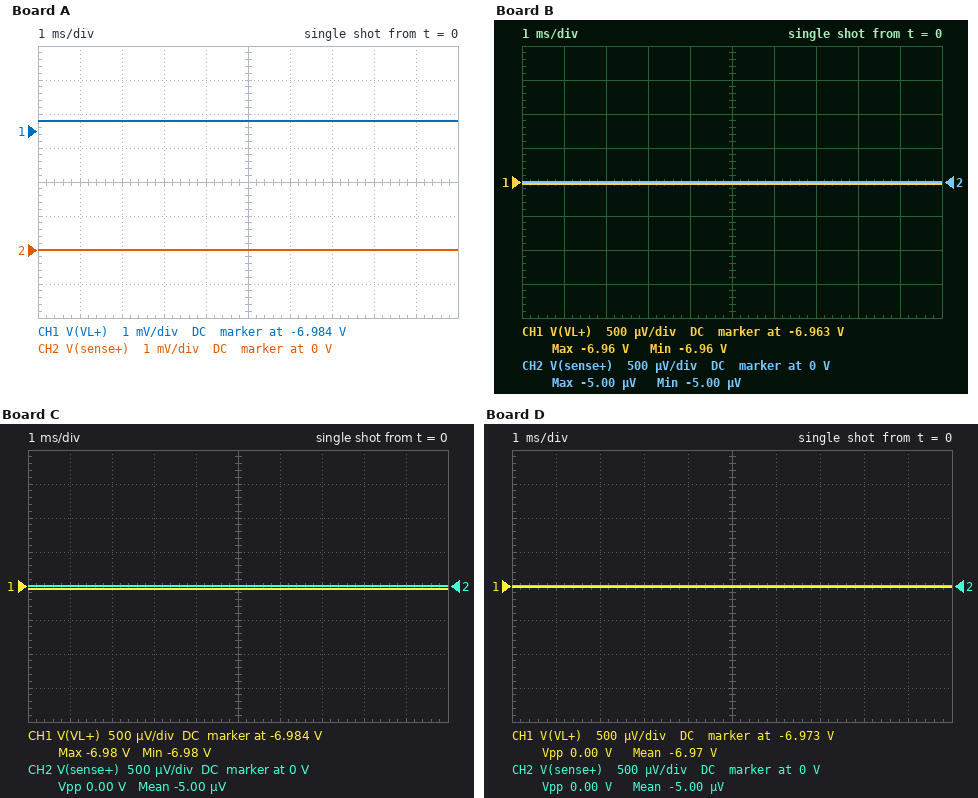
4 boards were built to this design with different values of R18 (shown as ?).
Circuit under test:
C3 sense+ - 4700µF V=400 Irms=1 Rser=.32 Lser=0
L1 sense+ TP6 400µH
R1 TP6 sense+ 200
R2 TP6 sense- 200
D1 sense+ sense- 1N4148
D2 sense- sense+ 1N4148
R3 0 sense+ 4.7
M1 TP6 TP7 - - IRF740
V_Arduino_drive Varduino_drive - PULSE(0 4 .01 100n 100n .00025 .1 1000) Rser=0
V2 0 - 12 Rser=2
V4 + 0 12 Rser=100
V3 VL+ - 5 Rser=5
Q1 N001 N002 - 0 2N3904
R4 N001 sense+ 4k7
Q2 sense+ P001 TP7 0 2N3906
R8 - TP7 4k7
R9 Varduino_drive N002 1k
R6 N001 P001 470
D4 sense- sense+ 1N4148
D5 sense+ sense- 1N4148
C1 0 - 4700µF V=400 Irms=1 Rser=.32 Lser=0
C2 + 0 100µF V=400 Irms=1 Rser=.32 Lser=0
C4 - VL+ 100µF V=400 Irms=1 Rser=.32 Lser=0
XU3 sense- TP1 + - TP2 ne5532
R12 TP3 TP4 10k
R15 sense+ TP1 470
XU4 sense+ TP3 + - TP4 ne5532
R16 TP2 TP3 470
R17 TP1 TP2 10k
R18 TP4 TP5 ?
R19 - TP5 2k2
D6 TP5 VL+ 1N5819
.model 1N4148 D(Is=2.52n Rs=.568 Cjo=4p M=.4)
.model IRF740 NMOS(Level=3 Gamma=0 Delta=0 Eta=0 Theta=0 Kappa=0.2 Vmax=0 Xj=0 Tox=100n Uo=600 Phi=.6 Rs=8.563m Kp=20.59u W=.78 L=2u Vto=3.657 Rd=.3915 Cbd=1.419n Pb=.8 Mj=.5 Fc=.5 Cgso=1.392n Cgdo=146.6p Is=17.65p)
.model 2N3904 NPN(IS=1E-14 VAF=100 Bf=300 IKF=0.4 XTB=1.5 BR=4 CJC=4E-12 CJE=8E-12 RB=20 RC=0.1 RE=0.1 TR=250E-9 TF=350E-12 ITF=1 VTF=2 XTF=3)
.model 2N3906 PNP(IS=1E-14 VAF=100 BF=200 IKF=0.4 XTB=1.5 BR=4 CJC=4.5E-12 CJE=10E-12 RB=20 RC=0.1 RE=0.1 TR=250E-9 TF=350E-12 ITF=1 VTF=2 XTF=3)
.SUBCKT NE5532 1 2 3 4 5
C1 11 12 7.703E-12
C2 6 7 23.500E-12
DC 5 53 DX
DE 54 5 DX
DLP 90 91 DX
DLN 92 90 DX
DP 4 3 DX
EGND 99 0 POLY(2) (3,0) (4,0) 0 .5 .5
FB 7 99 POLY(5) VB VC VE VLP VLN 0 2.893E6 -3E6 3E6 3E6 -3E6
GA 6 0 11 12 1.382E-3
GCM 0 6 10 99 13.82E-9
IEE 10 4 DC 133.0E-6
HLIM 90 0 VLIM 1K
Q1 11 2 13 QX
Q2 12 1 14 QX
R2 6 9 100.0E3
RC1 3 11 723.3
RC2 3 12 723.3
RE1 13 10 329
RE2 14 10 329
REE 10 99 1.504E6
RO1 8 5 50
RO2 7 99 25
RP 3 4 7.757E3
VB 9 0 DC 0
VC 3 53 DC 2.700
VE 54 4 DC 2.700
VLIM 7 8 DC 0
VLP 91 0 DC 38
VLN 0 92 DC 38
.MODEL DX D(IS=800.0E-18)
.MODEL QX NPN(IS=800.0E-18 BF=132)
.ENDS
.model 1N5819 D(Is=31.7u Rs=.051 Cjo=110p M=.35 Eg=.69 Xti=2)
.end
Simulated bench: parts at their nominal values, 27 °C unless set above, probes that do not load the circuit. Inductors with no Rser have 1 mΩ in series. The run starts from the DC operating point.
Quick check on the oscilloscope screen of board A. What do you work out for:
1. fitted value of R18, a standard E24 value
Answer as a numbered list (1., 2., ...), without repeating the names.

1. 3.9 kΩ
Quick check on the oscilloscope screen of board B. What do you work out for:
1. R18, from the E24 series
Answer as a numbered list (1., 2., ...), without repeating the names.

1. 1.3 kΩ
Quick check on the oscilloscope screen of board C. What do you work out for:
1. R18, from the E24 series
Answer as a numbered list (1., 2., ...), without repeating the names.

1. 5.6 kΩ
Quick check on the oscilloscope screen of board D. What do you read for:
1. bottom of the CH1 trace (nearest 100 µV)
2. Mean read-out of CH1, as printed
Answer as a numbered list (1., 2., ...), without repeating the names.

1. -6.9725 V
2. -6.97 V
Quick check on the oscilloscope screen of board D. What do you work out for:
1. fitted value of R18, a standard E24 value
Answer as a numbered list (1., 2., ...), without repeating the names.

1. 1.8 kΩ
